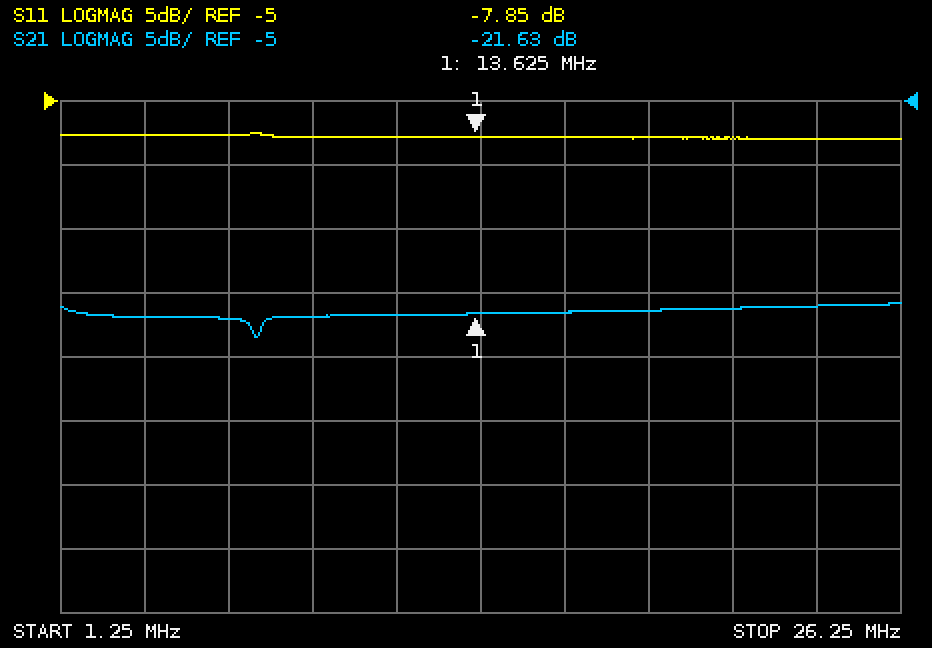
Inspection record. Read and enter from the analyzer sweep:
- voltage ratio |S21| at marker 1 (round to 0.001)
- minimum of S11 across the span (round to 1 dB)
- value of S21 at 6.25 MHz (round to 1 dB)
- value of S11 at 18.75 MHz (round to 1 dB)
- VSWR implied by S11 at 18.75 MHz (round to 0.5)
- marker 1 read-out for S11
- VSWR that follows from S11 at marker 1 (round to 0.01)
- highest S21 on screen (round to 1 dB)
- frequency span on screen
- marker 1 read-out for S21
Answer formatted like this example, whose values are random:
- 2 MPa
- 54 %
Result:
- 0.083
- -8 dB
- -22 dB
- -8 dB
- 2.5
- -7.85 dB
- 2.36
- -21 dB
- 25 MHz
- -21.63 dB
